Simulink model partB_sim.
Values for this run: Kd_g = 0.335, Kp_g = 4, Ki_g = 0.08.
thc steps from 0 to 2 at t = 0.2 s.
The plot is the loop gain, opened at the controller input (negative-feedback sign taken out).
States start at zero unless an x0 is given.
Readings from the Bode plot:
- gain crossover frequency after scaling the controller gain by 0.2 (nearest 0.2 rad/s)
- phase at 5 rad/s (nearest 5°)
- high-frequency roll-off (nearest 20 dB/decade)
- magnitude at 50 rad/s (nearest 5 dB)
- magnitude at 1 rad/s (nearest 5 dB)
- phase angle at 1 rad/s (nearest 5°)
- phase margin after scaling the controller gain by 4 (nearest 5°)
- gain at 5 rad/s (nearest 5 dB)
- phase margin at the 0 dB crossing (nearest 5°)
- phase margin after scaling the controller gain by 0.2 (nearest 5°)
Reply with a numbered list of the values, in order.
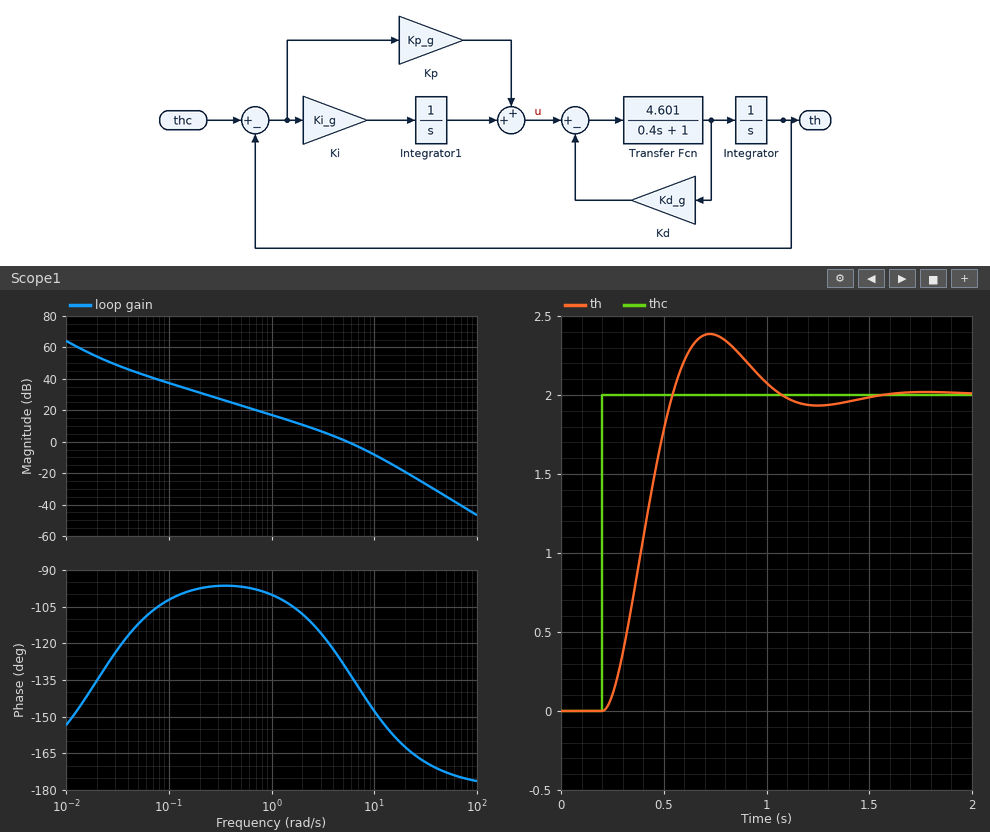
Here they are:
1. 1.4 rad/s
2. -130°
3. -40 dB/decade
4. -35 dB
5. 15 dB
6. -100°
7. 25°
8. 0 dB
9. 50°
10. 75°
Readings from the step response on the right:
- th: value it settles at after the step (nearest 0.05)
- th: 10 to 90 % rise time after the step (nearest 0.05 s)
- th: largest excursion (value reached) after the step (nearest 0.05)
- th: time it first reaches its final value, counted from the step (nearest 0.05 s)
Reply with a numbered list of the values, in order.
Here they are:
1. 2.00
2. 0.25 s
3. 2.40
4. 0.35 s
